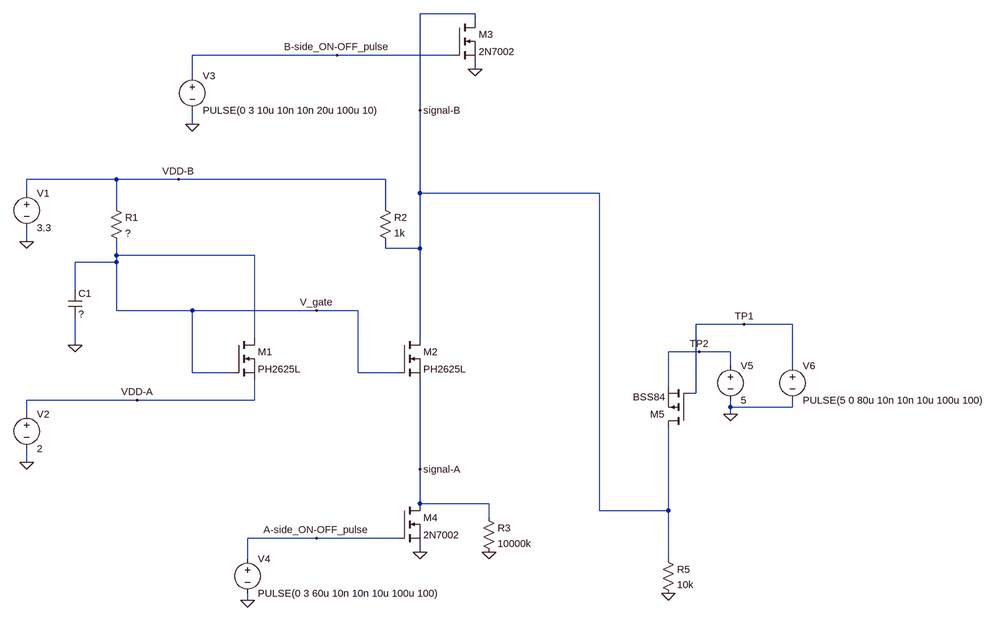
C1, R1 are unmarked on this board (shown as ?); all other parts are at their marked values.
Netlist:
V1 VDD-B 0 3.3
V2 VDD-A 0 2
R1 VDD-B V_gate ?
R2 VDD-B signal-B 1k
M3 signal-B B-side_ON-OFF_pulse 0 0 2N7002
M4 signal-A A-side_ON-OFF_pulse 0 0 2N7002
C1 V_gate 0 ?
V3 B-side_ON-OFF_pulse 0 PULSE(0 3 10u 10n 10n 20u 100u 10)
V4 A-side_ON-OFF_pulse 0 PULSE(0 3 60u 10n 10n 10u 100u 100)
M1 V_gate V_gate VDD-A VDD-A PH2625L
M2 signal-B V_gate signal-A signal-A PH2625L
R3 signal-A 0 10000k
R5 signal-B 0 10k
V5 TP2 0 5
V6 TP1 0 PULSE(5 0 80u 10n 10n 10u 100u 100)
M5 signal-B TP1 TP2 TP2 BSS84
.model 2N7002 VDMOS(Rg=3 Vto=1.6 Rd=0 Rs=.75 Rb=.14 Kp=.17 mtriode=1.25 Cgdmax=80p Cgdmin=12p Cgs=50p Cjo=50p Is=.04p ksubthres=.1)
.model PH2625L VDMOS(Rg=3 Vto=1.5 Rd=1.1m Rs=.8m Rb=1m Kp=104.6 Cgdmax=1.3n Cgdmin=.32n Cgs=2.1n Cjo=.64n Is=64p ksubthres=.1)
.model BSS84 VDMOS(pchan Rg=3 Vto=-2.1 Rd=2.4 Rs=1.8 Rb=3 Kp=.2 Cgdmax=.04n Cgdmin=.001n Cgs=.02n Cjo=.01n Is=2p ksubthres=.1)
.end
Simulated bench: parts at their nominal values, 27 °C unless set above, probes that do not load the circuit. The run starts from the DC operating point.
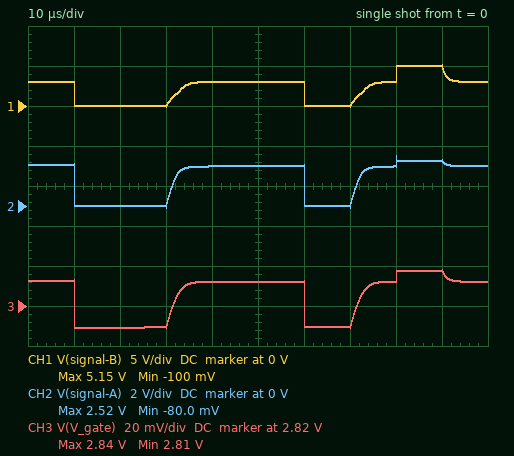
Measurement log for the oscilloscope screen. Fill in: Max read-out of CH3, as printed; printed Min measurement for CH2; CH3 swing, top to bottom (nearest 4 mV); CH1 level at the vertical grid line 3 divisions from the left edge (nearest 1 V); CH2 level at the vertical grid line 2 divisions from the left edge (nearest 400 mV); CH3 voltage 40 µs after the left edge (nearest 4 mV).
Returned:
2.84 V
-80.0 mV
28 mV
0 V
0 V
2.832 V
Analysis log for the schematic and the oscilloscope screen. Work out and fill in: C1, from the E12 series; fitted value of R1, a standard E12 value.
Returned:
330 nF
560 kΩ
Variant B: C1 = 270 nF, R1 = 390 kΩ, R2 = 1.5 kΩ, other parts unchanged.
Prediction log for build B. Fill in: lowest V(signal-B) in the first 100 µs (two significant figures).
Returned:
-86 mV
